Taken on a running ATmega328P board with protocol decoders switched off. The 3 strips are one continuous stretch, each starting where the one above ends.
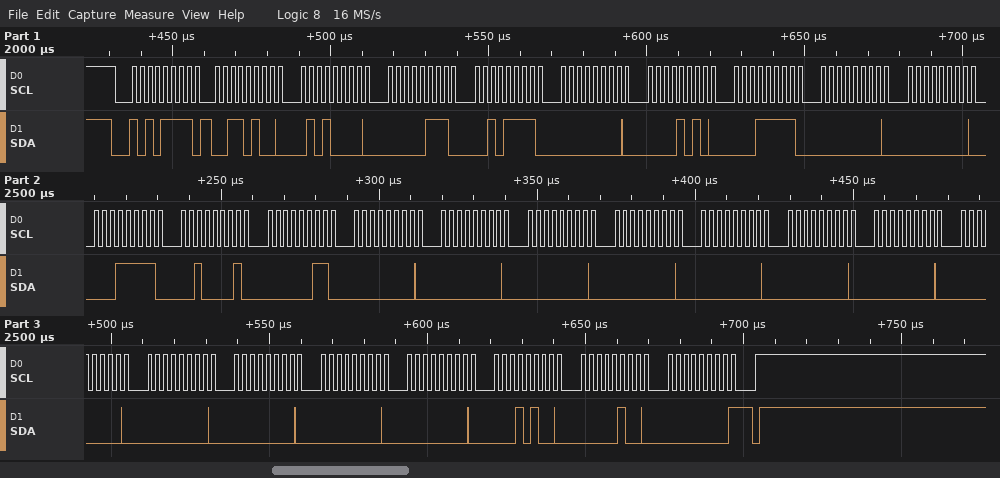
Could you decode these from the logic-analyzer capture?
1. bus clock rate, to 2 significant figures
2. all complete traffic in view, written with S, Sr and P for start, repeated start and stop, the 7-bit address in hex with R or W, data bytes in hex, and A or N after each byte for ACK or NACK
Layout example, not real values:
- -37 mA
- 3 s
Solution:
- 400 kHz
- S 57R A 34 A 50 A 07 A 2F A 00 A 0A A 1F A 00 A 00 A 1F A 21 A 03 A 00 A 00 A 00 A 00 A 00 A 00 A 00 A 00 A 00 A 00 A 00 A 00 A 14 A 04 A 00 N P
